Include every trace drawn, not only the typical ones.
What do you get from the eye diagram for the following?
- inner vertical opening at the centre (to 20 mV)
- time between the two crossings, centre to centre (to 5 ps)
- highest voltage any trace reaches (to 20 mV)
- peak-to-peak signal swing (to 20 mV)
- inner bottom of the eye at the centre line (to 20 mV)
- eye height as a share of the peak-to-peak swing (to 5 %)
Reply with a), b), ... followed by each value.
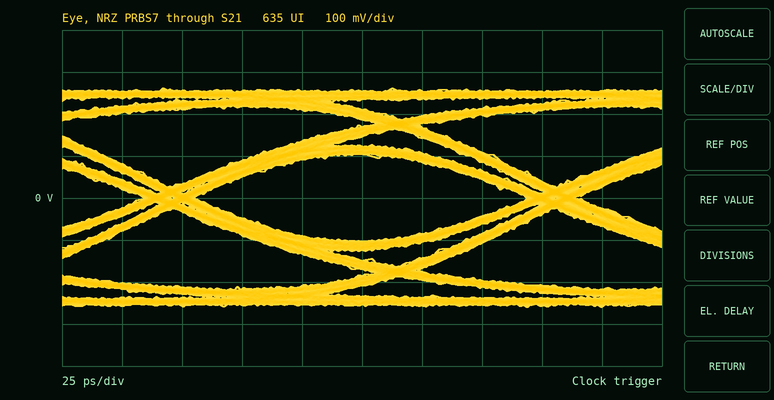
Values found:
a) 200 mV
b) 160 ps
c) 260 mV
d) 520 mV
e) -100 mV
f) 40 %
